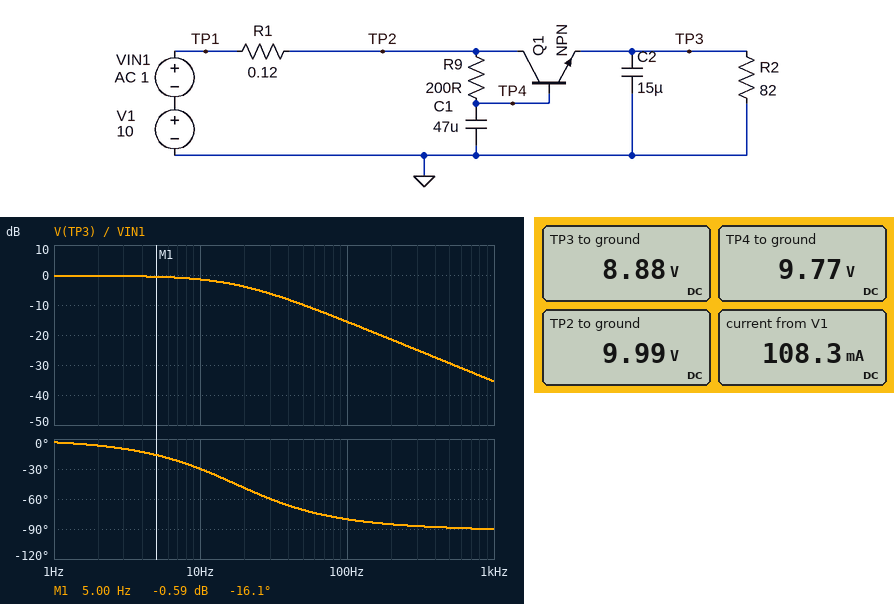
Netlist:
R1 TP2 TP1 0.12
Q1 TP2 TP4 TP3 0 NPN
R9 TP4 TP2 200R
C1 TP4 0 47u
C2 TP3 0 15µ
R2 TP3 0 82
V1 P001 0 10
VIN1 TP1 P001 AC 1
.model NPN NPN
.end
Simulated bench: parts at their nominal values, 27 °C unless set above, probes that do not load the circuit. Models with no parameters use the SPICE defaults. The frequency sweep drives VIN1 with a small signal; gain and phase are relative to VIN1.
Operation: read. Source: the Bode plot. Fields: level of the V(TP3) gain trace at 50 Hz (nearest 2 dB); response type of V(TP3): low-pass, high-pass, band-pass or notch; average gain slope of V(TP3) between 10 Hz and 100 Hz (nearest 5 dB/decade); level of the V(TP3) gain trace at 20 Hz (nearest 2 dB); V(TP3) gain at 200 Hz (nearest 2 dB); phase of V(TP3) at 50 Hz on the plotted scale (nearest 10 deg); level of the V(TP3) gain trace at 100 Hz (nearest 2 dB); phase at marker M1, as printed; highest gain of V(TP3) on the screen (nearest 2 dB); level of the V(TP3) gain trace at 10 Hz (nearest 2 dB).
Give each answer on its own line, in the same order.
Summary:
-10 dB
low-pass
-15 dB/decade
-4 dB
-22 dB
-70 deg
-16 dB
-16.1 deg
0 dB
-2 dB
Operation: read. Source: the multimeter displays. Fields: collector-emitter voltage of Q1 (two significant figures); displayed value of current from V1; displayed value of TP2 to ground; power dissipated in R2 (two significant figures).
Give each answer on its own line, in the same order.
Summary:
1.1 V
108.3 mA
9.99 V
960 mW
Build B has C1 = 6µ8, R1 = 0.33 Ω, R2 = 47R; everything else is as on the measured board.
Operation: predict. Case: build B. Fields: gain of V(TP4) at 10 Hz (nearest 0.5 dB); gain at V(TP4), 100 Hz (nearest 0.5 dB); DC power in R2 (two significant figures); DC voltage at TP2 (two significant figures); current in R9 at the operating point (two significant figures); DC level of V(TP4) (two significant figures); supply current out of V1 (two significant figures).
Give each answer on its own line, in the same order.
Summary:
-0.5 dB
-2.5 dB
1.6 W
9.9 V
1.8 mA
9.6 V
180 mA
